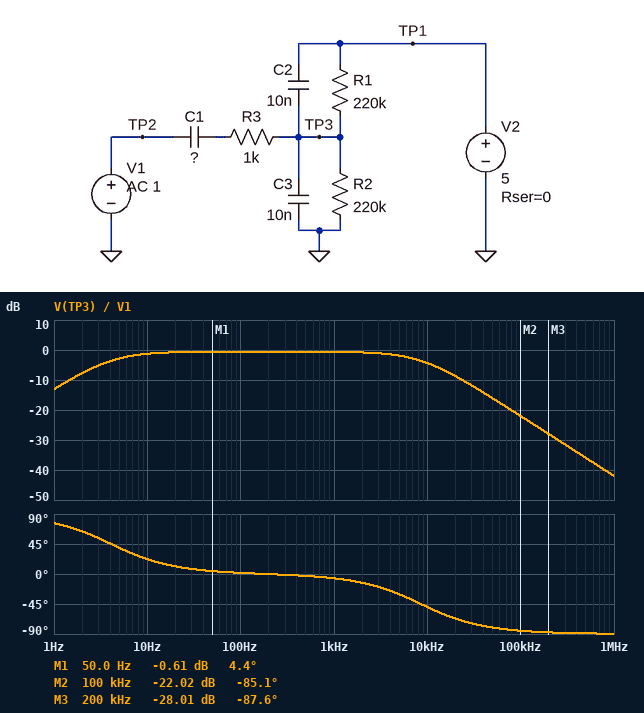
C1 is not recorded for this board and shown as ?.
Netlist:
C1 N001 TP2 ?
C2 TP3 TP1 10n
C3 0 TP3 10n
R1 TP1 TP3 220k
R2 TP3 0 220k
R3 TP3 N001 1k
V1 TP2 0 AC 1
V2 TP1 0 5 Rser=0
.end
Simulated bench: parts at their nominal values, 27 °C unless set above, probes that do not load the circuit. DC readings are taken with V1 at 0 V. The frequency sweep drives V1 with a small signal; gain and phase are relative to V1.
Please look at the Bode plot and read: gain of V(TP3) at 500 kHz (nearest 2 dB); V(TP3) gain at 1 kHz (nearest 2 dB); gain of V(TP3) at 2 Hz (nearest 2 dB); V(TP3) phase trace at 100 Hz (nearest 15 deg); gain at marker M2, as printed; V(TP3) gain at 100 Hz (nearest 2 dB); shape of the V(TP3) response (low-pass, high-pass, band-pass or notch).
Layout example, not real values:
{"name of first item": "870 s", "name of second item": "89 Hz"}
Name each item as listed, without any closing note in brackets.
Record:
{"gain of V(TP3) at 500 kHz": "-36 dB", "V(TP3) gain at 1 kHz": "0 dB", "gain of V(TP3) at 2 Hz": "-8 dB", "V(TP3) phase trace at 100 Hz": "0 deg", "gain at marker M2, as printed": "-22.02 dB", "V(TP3) gain at 100 Hz": "0 dB", "shape of the V(TP3) response": "band-pass"}
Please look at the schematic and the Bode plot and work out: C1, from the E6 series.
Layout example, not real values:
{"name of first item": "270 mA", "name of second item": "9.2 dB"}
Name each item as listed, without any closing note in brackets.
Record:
{"C1, from the E6 series": "330 nF"}
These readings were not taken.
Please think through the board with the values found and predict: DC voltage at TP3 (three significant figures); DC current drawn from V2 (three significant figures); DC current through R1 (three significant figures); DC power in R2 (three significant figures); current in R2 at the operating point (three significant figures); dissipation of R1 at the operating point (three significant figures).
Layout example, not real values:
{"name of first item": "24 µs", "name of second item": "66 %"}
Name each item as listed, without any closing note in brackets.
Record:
{"DC voltage at TP3": "2.50 V", "DC current drawn from V2": "11.4 µA", "DC current through R1": "11.4 µA", "DC power in R2": "28.4 µW", "current in R2 at the operating point": "11.4 µA", "dissipation of R1 at the operating point": "28.4 µW"}
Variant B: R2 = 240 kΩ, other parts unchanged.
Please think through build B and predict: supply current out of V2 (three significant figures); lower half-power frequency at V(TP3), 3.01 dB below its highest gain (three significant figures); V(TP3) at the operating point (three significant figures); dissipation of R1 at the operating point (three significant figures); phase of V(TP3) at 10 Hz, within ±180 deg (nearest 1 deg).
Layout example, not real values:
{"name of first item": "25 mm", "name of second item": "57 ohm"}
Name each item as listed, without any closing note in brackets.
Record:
{"supply current out of V2": "10.9 µA", "lower half-power frequency at V(TP3), 3.01 dB below its highest gain": "3.93 Hz", "V(TP3) at the operating point": "2.61 V", "dissipation of R1 at the operating point": "26.0 µW", "phase of V(TP3) at 10 Hz, within ±180 deg": "21 deg"}
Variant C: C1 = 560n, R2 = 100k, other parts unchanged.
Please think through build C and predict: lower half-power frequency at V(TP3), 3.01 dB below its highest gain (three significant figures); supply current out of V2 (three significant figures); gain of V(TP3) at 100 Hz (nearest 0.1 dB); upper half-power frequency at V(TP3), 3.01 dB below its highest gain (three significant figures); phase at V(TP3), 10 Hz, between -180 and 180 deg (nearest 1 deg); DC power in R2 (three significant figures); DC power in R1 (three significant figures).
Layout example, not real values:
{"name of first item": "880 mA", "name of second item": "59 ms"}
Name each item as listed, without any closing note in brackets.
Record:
{"lower half-power frequency at V(TP3), 3.01 dB below its highest gain": "3.93 Hz", "supply current out of V2": "15.6 µA", "gain of V(TP3) at 100 Hz": "-0.4 dB", "upper half-power frequency at V(TP3), 3.01 dB below its highest gain": "8.36 kHz", "phase at V(TP3), 10 Hz, between -180 and 180 deg": "21 deg", "DC power in R2": "24.4 µW", "DC power in R1": "53.7 µW"}
